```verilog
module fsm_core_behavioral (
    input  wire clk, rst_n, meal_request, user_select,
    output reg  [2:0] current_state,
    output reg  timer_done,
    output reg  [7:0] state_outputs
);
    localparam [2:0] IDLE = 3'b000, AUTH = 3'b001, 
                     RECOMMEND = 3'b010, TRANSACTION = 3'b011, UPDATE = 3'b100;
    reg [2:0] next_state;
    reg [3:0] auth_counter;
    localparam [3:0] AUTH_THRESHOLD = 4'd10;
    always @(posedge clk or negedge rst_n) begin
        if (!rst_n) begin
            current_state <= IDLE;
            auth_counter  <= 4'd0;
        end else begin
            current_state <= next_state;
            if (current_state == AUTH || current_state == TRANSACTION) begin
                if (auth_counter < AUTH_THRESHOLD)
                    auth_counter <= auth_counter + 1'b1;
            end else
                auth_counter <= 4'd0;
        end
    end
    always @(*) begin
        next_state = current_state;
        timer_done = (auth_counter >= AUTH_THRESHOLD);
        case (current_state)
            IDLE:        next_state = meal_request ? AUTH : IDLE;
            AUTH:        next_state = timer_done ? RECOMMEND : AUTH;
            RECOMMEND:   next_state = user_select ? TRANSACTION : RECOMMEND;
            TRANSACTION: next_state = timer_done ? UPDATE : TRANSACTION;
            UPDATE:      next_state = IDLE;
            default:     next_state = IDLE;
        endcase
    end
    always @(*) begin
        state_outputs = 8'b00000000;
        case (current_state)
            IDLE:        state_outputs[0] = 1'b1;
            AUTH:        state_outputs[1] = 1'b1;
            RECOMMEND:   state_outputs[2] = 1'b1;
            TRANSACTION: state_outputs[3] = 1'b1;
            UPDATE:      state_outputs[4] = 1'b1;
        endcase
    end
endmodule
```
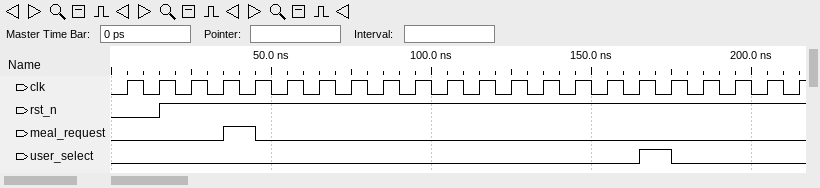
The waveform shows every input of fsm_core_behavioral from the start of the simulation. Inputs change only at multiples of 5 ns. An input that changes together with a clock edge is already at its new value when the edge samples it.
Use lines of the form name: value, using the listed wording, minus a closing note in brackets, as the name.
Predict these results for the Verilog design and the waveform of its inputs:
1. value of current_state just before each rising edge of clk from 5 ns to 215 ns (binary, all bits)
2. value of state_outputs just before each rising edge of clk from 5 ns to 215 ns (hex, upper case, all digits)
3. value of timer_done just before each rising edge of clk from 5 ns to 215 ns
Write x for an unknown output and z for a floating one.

value of current_state just before each rising edge of clk from 5 ns to 215 ns: 000, 000, 000, 000, 001, 001, 001, 001, 001, 001, 001, 001, 001, 001, 001, 010, 010, 011, 011, 011, 011, 011
value of state_outputs just before each rising edge of clk from 5 ns to 215 ns: 01, 01, 01, 01, 02, 02, 02, 02, 02, 02, 02, 02, 02, 02, 02, 04, 04, 08, 08, 08, 08, 08
value of timer_done just before each rising edge of clk from 5 ns to 215 ns: 0 0 0 0 0 0 0 0 0 0 0 0 0 0 1 1 0 0 0 0 0 0
